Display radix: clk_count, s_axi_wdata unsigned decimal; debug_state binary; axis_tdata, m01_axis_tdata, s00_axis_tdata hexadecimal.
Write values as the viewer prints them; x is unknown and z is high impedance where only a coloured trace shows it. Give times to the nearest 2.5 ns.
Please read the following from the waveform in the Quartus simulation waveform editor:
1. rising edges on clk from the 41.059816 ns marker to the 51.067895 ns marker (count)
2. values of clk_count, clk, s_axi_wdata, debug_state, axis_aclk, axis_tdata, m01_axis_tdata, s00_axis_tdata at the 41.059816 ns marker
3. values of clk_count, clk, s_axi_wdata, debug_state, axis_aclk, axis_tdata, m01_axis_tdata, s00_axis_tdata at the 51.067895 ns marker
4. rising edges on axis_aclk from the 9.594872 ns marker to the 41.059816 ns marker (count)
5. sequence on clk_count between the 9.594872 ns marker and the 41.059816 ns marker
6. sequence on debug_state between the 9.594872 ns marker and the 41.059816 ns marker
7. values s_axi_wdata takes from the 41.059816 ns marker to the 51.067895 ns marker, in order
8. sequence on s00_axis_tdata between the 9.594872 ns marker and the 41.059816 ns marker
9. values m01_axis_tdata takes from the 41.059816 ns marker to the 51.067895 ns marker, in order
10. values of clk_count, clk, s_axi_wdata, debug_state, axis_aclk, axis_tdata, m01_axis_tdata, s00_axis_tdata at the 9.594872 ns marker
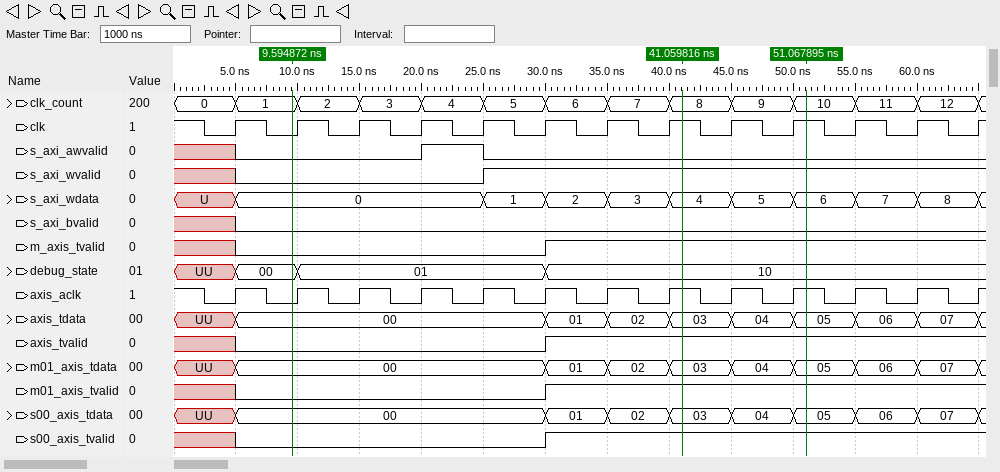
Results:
2
clk_count=8, clk=1, s_axi_wdata=4, debug_state=10, axis_aclk=1, axis_tdata=03, m01_axis_tdata=03, s00_axis_tdata=03
clk_count=10, clk=1, s_axi_wdata=6, debug_state=10, axis_aclk=1, axis_tdata=05, m01_axis_tdata=05, s00_axis_tdata=05
7
1, 2, 3, 4, 5, 6, 7, 8
00, 01, 10
4, 5, 6
00, 01, 02, 03
03, 04, 05
clk_count=1, clk=0, s_axi_wdata=0, debug_state=00, axis_aclk=0, axis_tdata=00, m01_axis_tdata=00, s00_axis_tdata=00
